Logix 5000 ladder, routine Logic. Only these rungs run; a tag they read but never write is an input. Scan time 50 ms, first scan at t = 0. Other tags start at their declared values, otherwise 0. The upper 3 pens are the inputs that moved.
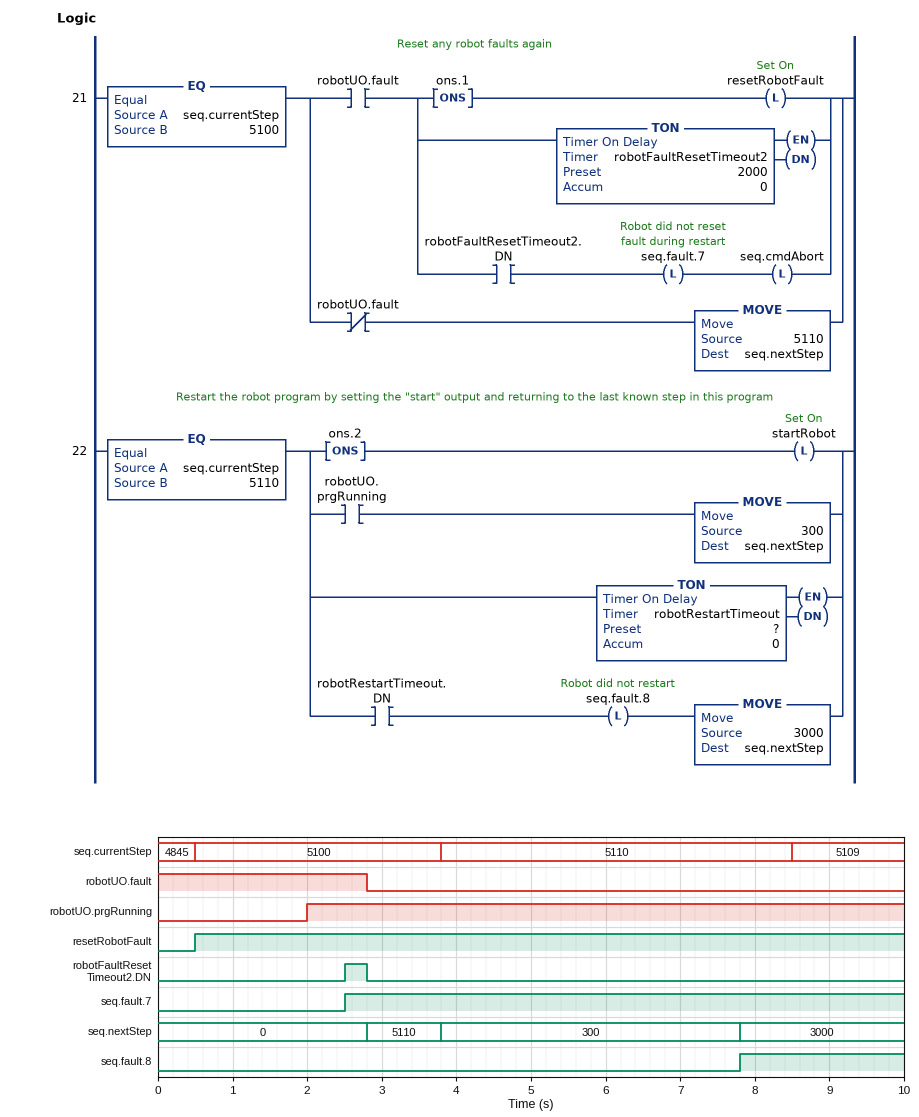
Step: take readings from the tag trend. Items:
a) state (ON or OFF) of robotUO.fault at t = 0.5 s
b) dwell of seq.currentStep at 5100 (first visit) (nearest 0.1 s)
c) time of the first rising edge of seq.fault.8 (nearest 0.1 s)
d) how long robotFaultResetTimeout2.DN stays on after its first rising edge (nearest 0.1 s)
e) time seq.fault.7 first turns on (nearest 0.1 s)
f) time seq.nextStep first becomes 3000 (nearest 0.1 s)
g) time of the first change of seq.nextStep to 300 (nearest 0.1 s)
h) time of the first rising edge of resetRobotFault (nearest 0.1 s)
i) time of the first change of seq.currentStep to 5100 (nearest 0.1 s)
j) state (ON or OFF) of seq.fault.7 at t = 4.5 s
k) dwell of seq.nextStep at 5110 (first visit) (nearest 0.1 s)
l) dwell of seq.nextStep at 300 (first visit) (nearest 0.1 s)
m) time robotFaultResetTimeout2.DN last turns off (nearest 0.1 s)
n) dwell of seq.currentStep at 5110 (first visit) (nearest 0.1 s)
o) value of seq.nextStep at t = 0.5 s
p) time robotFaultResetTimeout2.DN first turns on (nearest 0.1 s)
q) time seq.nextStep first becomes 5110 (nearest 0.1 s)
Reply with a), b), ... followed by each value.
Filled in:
a) ON
b) 3.3 s
c) 7.8 s
d) 0.3 s
e) 2.5 s
f) 7.8 s
g) 3.8 s
h) 0.5 s
i) 0.5 s
j) ON
k) 1.0 s
l) 4.0 s
m) 2.8 s
n) 4.7 s
o) 0
p) 2.5 s
q) 2.8 s
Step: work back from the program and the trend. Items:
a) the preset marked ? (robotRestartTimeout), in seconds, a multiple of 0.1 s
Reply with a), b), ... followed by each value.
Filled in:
a) 4.0 s
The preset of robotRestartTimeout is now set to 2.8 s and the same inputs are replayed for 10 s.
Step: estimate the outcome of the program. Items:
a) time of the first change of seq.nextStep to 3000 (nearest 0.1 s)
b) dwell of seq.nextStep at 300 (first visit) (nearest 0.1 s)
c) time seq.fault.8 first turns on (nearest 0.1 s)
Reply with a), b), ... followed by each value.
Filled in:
a) 6.6 s
b) 2.8 s
c) 6.6 s
